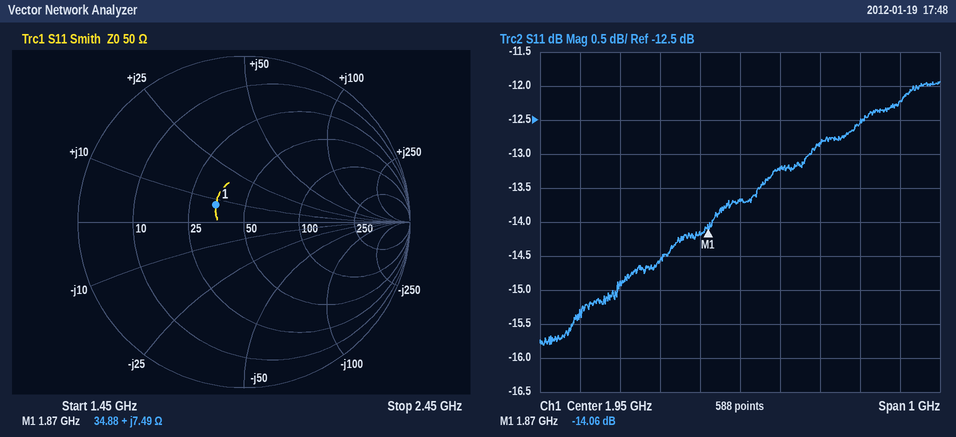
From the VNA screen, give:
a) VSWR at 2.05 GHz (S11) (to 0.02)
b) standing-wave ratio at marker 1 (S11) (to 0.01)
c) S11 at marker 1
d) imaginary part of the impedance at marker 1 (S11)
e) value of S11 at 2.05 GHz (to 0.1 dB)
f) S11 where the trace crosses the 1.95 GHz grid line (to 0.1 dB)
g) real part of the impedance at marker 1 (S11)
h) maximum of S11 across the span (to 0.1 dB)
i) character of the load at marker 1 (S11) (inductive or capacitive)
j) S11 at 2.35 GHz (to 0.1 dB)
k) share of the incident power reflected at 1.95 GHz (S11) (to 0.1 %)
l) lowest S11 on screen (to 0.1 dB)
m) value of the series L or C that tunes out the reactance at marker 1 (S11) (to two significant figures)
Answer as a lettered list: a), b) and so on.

a) 1.56
b) 1.49
c) -14.06 dB
d) +7.49 Ω
e) -13.2 dB
f) -13.7 dB
g) 34.88 Ω
h) -11.9 dB
i) inductive
j) -12.2 dB
k) 4.3 %
l) -15.8 dB
m) 11 pF
